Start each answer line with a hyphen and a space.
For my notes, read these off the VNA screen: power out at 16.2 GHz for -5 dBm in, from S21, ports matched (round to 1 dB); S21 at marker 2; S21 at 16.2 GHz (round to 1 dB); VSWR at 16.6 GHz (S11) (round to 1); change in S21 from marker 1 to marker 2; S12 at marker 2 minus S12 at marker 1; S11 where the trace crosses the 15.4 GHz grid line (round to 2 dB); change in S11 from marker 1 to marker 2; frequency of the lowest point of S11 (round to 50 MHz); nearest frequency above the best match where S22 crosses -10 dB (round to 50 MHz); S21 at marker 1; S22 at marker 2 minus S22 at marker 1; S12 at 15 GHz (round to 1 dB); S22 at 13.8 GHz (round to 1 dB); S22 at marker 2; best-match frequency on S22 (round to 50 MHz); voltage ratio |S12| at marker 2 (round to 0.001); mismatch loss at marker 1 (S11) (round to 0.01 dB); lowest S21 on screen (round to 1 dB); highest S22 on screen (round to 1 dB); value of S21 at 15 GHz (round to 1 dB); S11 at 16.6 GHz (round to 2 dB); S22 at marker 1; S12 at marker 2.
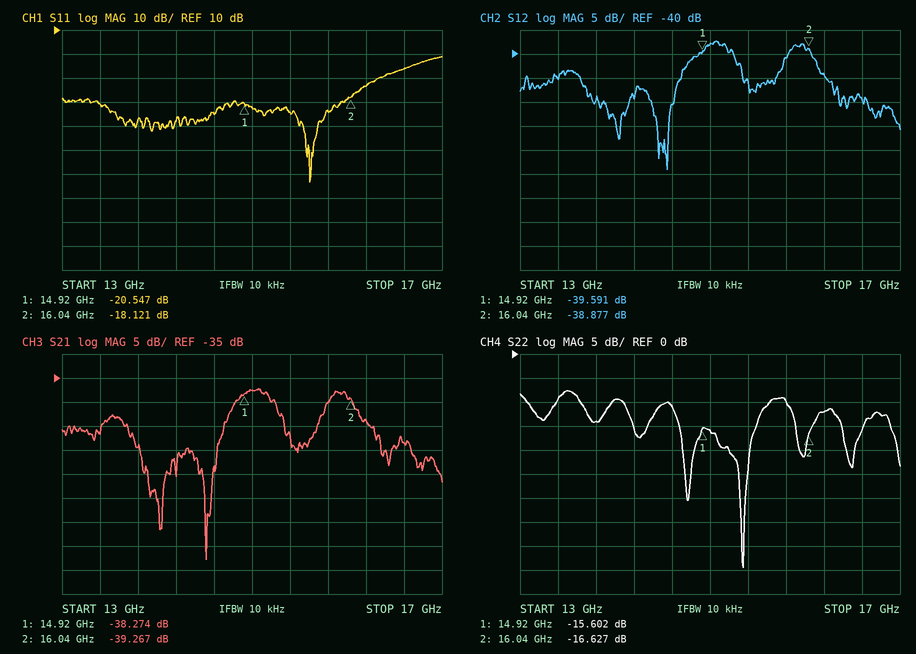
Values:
- -49 dBm
- -39.267 dB
- -44 dB
- 3
- -0.993 dB
- 0.714 dB
- -24 dB
- 2.426 dB
- 15.60 GHz
- 15.65 GHz
- -38.274 dB
- -1.025 dB
- -38 dB
- -14 dB
- -16.627 dB
- 15.35 GHz
- 0.011
- 0.04 dB
- -73 dB
- -8 dB
- -38 dB
- -6 dB
- -15.602 dB
- -38.877 dB
